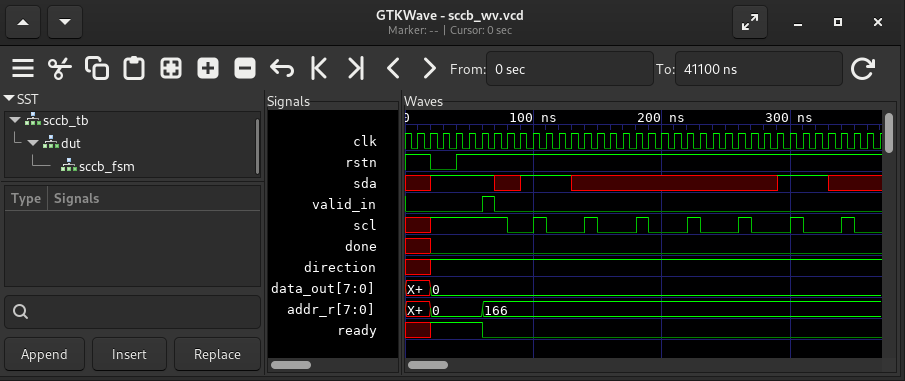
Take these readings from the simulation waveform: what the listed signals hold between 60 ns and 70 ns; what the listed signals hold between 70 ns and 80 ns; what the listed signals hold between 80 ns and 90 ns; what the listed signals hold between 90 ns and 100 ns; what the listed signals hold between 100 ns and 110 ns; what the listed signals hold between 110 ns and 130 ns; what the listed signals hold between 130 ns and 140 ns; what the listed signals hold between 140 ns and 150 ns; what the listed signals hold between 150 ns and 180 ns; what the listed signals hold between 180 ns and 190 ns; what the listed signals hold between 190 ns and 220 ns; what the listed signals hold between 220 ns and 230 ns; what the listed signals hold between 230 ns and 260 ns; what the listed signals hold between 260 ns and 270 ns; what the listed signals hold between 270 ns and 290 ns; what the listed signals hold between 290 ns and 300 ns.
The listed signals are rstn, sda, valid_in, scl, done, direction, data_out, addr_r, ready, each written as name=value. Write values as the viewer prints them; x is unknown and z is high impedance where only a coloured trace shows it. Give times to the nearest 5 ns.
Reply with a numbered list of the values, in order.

1. rstn=1, sda=1, valid_in=1, scl=1, done=0, direction=1, data_out=0, addr_r=166, ready=0
2. rstn=1, sda=x, valid_in=0, scl=1, done=0, direction=1, data_out=0, addr_r=166, ready=0
3. rstn=1, sda=x, valid_in=0, scl=0, done=0, direction=1, data_out=0, addr_r=166, ready=0
4. rstn=1, sda=1, valid_in=0, scl=0, done=0, direction=1, data_out=0, addr_r=166, ready=0
5. rstn=1, sda=1, valid_in=0, scl=1, done=0, direction=1, data_out=0, addr_r=166, ready=0
6. rstn=1, sda=1, valid_in=0, scl=0, done=0, direction=1, data_out=0, addr_r=166, ready=0
7. rstn=1, sda=x, valid_in=0, scl=0, done=0, direction=1, data_out=0, addr_r=166, ready=0
8. rstn=1, sda=x, valid_in=0, scl=1, done=0, direction=1, data_out=0, addr_r=166, ready=0
9. rstn=1, sda=x, valid_in=0, scl=0, done=0, direction=1, data_out=0, addr_r=166, ready=0
10. rstn=1, sda=x, valid_in=0, scl=1, done=0, direction=1, data_out=0, addr_r=166, ready=0
11. rstn=1, sda=x, valid_in=0, scl=0, done=0, direction=1, data_out=0, addr_r=166, ready=0
12. rstn=1, sda=x, valid_in=0, scl=1, done=0, direction=1, data_out=0, addr_r=166, ready=0
13. rstn=1, sda=x, valid_in=0, scl=0, done=0, direction=1, data_out=0, addr_r=166, ready=0
14. rstn=1, sda=x, valid_in=0, scl=1, done=0, direction=1, data_out=0, addr_r=166, ready=0
15. rstn=1, sda=x, valid_in=0, scl=0, done=0, direction=1, data_out=0, addr_r=166, ready=0
16. rstn=1, sda=1, valid_in=0, scl=0, done=0, direction=1, data_out=0, addr_r=166, ready=0
